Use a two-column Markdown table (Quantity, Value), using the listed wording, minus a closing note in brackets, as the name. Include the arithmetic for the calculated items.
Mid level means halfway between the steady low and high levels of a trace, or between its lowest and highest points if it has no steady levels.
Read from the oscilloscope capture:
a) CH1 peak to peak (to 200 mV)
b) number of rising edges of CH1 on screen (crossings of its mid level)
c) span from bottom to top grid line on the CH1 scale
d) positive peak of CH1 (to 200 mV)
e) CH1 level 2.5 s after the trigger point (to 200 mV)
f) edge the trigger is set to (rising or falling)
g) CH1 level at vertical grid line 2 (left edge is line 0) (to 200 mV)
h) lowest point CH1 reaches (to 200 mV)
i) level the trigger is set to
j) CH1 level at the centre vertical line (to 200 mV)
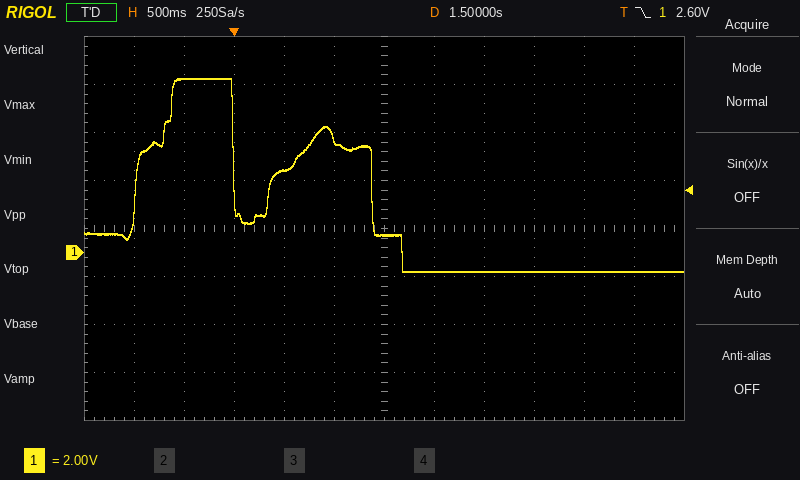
| Quantity | Value |
|---|---|
| CH1 peak to peak | 7.2 V − (-800 mV) = 8.0 V |
| number of rising edges of CH1 on screen | 2 |
| span from bottom to top grid line on the CH1 scale | 16 V |
| positive peak of CH1 | 7.2 V |
| CH1 level 2.5 s after the trigger point | -800 mV |
| edge the trigger is set to | falling |
| CH1 level at vertical grid line 2 (left edge is line 0) | 7.2 V |
| lowest point CH1 reaches | -800 mV |
| level the trigger is set to | 2.60 V |
| CH1 level at the centre vertical line | 800 mV |
